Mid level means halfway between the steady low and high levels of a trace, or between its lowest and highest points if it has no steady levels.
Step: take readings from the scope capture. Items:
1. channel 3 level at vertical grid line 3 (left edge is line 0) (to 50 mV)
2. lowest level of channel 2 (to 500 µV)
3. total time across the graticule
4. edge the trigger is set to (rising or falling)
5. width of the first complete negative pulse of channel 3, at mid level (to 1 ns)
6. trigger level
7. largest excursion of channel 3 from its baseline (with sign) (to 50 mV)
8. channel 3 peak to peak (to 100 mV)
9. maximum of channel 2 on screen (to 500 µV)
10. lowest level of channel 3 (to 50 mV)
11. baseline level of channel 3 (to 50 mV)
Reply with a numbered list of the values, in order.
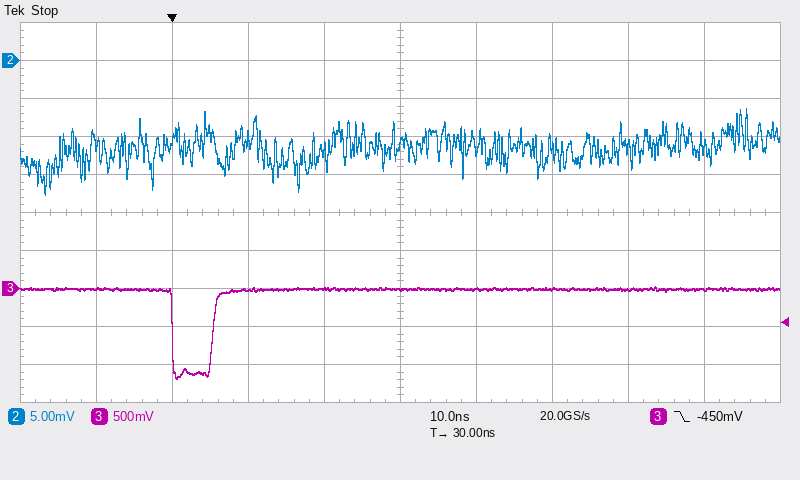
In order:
1. 0 mV
2. -17.5 mV
3. 100 ns
4. falling
5. 5 ns
6. -450 mV
7. -1.20 V
8. 1.20 V
9. -6.5 mV
10. -1.20 V
11. 0 mV
